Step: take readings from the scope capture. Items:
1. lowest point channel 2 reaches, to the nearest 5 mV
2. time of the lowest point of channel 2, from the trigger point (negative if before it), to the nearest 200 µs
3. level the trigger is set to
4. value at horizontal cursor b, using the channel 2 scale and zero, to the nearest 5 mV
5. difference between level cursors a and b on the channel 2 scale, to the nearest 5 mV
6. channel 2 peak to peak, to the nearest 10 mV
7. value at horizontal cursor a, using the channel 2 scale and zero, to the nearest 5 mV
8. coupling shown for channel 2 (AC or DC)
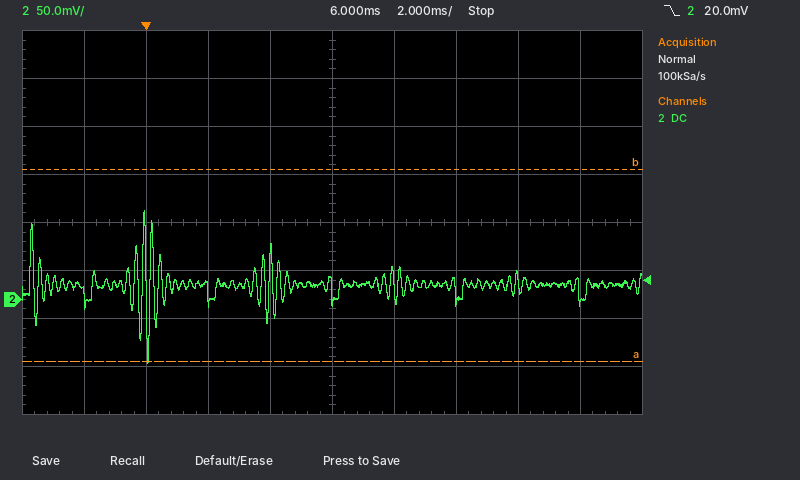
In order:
-65 mV
0.0 ms
20.0 mV
135 mV
200 mV
160 mV
-65 mV
DC
